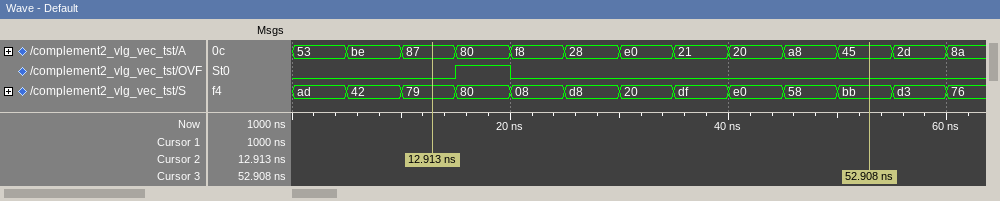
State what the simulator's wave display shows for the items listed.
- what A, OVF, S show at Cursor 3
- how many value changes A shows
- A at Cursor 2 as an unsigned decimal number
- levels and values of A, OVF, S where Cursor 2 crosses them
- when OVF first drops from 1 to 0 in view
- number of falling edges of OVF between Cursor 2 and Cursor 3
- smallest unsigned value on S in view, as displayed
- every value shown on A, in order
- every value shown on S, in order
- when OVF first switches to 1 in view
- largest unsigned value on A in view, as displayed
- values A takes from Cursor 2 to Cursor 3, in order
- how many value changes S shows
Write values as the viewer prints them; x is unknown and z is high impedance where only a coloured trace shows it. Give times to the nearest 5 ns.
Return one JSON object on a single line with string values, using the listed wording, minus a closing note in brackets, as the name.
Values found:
{"what A, OVF, S show at Cursor 3": "A=45, OVF=0, S=bb", "how many value changes A shows": "12", "A at Cursor 2 as an unsigned decimal number": "135", "levels and values of A, OVF, S where Cursor 2 crosses them": "A=87, OVF=0, S=79", "when OVF first drops from 1 to 0 in view": "20 ns", "number of falling edges of OVF between Cursor 2 and Cursor 3": "1", "smallest unsigned value on S in view, as displayed": "08", "every value shown on A, in order": "53, be, 87, 80, f8, 28, e0, 21, 20, a8, 45, 2d, 8a", "every value shown on S, in order": "ad, 42, 79, 80, 08, d8, 20, df, e0, 58, bb, d3, 76", "when OVF first switches to 1 in view": "15 ns", "largest unsigned value on A in view, as displayed": "f8", "values A takes from Cursor 2 to Cursor 3, in order": "87, 80, f8, 28, e0, 21, 20, a8, 45", "how many value changes S shows": "12"}
